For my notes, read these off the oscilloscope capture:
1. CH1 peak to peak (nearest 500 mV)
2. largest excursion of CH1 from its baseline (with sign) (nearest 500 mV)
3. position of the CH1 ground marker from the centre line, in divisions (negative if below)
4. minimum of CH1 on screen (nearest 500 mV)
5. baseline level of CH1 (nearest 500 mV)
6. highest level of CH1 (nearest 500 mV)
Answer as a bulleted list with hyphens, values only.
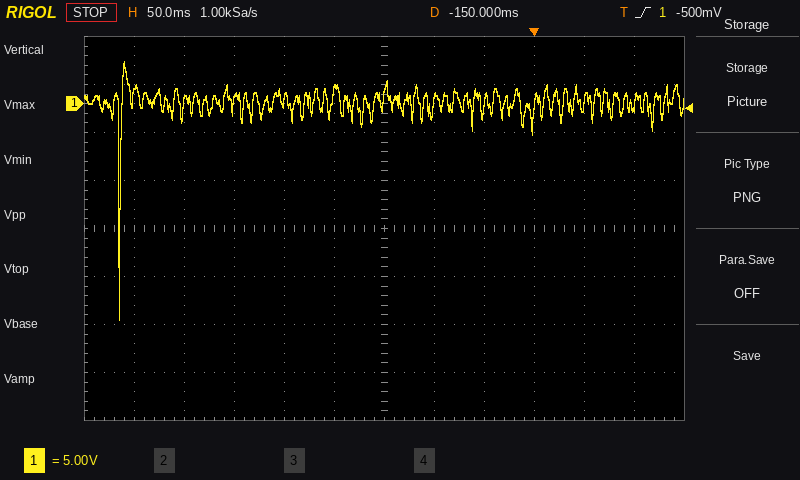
- 27.0 V
- -23.0 V
- +2.6 div
- -22.5 V
- 500 mV
- 4.5 V
